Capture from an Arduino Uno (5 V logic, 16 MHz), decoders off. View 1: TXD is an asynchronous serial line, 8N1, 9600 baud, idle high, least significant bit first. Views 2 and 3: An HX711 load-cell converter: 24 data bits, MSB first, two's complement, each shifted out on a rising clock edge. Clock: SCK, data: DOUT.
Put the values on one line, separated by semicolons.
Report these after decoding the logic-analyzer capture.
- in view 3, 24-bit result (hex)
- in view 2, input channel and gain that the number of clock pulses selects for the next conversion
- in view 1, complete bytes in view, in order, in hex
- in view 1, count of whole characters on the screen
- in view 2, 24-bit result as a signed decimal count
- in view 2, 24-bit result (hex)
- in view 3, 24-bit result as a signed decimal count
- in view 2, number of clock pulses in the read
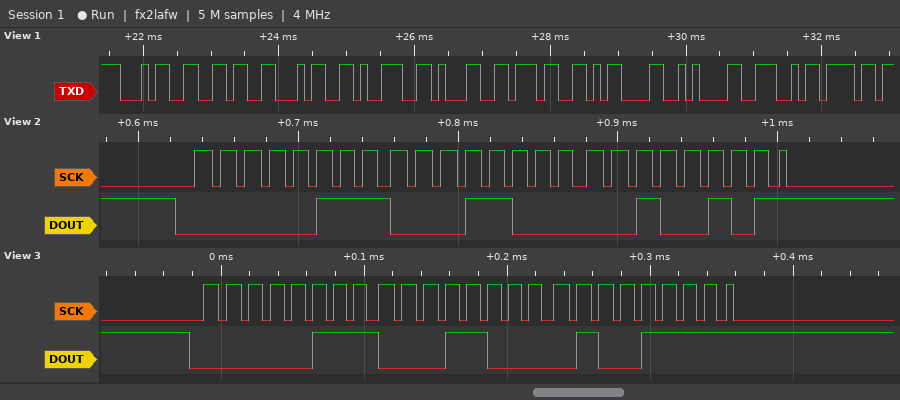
0x07184F; channel A, gain 128; 34 36 34 39 31 37 0D 0A 4E 6F; 10; 464933; 0x071825; 464975; 25
